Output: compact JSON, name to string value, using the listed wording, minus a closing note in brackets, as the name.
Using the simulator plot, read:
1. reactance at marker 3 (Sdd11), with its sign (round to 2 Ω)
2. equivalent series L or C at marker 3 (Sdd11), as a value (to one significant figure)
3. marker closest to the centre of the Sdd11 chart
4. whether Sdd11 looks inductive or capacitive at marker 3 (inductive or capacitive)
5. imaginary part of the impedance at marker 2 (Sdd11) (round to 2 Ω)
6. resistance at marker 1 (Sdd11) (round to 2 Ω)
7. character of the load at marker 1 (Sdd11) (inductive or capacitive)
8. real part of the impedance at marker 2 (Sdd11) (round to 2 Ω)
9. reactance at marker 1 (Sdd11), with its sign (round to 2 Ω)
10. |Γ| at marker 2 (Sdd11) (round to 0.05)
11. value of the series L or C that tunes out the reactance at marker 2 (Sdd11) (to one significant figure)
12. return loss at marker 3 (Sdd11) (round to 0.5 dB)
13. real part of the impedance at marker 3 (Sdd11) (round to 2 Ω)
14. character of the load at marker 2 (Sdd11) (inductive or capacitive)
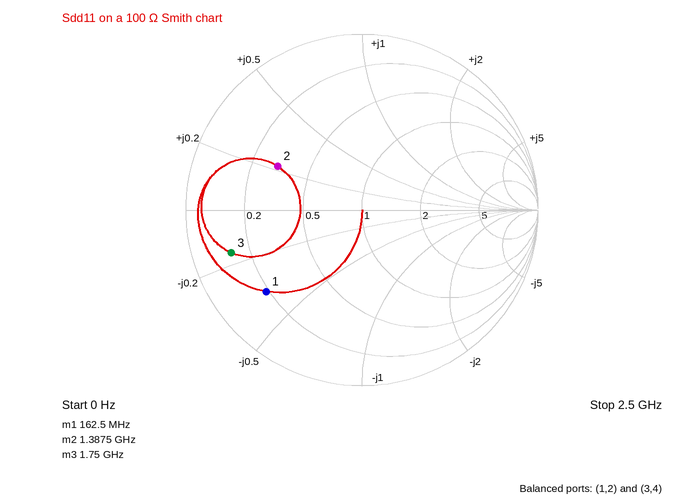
{"reactance at marker 3 (Sdd11), with its sign": "-16 Ω", "equivalent series L or C at marker 3 (Sdd11), as a value": "6 pF", "marker closest to the centre of the Sdd11 chart": "marker 2", "whether Sdd11 looks inductive or capacitive at marker 3": "capacitive", "imaginary part of the impedance at marker 2 (Sdd11)": "+22 Ω", "resistance at marker 1 (Sdd11)": "18 Ω", "character of the load at marker 1 (Sdd11)": "capacitive", "real part of the impedance at marker 2 (Sdd11)": "32 Ω", "reactance at marker 1 (Sdd11), with its sign": "-36 Ω", "|Γ| at marker 2 (Sdd11)": "0.55", "value of the series L or C that tunes out the reactance at marker 2 (Sdd11)": "5 pF", "return loss at marker 3 (Sdd11)": "2.0 dB", "real part of the impedance at marker 3 (Sdd11)": "12 Ω", "character of the load at marker 2 (Sdd11)": "inductive"}
